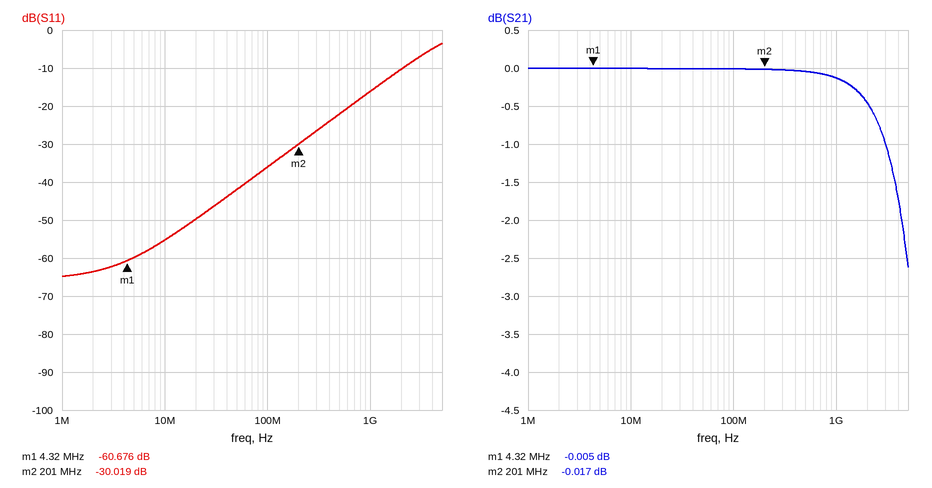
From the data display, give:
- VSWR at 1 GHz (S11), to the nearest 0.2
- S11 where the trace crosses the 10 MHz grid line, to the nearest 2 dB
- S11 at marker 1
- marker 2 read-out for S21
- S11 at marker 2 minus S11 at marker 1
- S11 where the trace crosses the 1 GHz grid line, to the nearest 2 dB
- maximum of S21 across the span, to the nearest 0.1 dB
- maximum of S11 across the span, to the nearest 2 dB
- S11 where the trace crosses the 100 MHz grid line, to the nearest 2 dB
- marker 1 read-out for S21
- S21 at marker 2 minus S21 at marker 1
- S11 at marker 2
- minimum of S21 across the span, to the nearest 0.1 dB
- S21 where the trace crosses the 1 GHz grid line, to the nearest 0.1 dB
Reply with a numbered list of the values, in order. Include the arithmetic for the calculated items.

1. |Γ| = 10^(-16/20) = 0.1585; VSWR = (1 + 0.1585)/(1 − 0.1585) ≈ 1.4
2. -56 dB
3. -60.676 dB
4. -0.017 dB
5. -30.019 − (-60.676) = 30.657 dB
6. -16 dB
7. 0.0 dB
8. -4 dB
9. -36 dB
10. -0.005 dB
11. -0.017 − (-0.005) = -0.012 dB
12. -30.019 dB
13. -2.6 dB
14. -0.1 dB
